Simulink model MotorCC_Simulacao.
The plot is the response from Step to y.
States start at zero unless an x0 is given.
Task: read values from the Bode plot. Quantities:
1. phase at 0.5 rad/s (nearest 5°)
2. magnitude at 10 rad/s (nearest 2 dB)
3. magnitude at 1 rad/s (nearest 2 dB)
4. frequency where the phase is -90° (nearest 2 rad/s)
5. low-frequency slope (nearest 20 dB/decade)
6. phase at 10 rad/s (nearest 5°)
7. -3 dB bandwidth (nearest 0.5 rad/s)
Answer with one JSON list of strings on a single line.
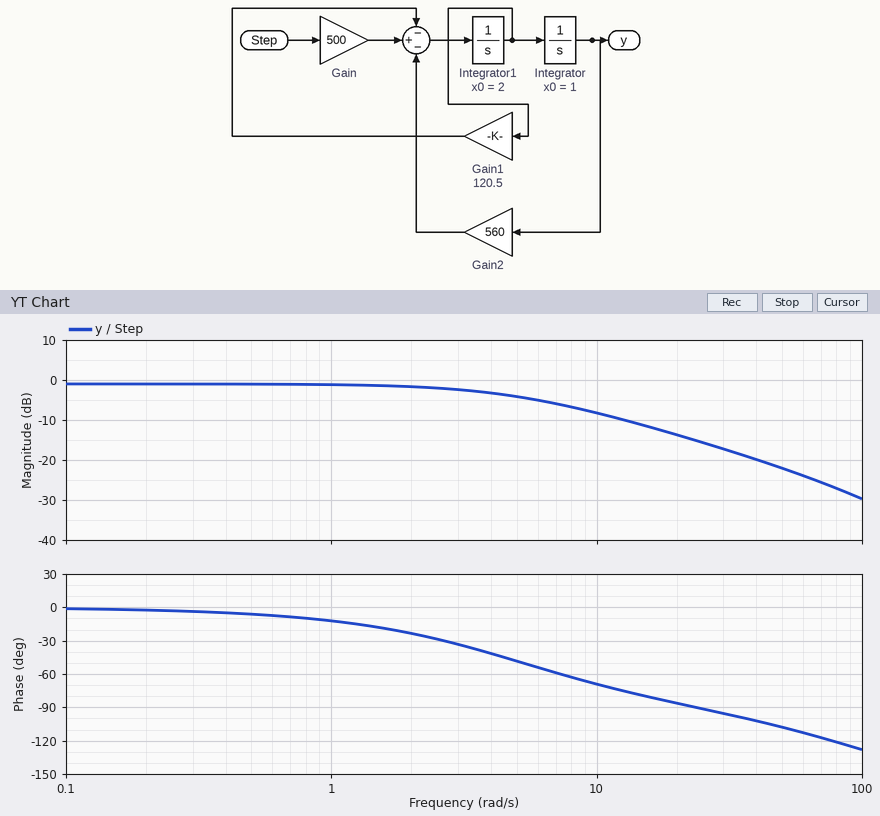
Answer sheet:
["-5°", "-8 dB", "-2 dB", "24 rad/s", "0 dB/decade", "-70°", "5.0 rad/s"]
